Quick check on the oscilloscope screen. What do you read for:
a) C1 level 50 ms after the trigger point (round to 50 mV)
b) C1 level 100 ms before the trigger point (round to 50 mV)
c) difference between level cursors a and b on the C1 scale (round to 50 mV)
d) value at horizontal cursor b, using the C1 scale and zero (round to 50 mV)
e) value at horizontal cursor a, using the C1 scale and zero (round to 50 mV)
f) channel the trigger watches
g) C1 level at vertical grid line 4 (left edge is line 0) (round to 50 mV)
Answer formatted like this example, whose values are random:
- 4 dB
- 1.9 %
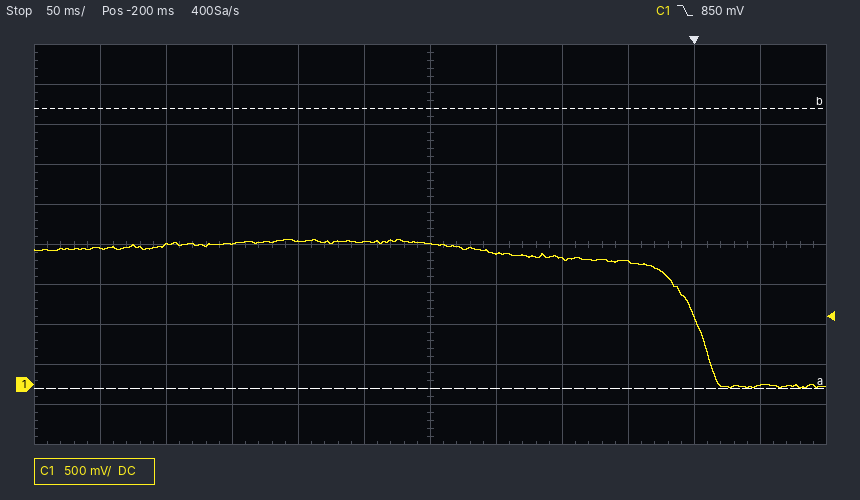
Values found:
- 0 mV
- 1.55 V
- 3.50 V
- 3.45 V
- -50 mV
- C1
- 1.80 V
